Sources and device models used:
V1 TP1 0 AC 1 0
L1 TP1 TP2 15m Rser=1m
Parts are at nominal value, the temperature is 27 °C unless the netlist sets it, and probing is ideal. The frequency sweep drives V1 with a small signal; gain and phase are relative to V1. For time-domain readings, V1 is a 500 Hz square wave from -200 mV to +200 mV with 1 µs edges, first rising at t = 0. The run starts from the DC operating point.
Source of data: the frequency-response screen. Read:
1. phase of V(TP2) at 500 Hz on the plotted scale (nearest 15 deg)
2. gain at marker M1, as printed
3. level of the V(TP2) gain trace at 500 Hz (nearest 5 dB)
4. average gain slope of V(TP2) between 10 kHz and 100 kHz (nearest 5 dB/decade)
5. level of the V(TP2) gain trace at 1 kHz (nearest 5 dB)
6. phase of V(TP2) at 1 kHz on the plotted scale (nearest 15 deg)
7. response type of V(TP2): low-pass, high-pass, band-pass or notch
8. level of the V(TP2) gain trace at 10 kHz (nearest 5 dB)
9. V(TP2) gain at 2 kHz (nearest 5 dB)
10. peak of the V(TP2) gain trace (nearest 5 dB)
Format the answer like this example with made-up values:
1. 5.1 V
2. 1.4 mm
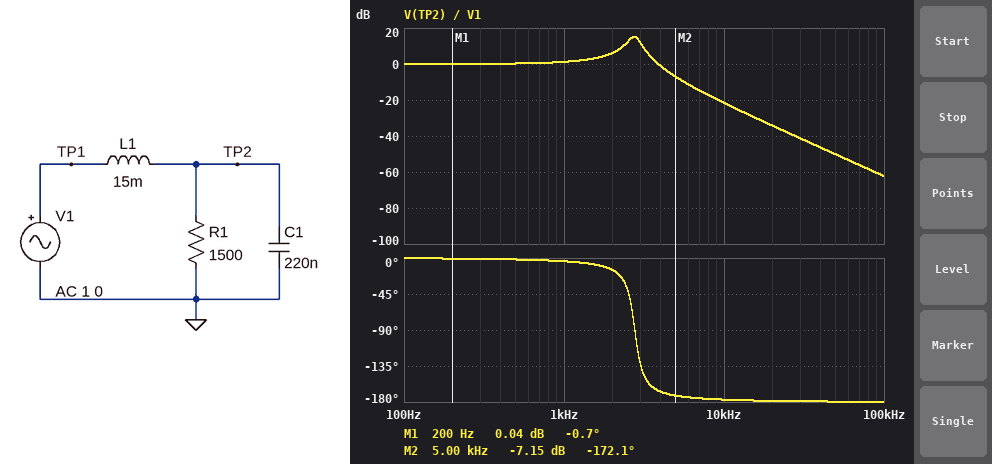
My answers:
1. 0 deg
2. 0.04 dB
3. 0 dB
4. -40 dB/decade
5. 0 dB
6. 0 deg
7. low-pass
8. -20 dB
9. 5 dB
10. 15 dB
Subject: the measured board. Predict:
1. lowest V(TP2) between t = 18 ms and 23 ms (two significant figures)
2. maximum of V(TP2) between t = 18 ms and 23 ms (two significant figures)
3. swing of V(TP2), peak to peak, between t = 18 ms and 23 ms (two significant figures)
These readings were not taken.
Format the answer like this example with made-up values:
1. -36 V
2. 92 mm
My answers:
1. -500 mV
2. 500 mV
3. 1.0 V
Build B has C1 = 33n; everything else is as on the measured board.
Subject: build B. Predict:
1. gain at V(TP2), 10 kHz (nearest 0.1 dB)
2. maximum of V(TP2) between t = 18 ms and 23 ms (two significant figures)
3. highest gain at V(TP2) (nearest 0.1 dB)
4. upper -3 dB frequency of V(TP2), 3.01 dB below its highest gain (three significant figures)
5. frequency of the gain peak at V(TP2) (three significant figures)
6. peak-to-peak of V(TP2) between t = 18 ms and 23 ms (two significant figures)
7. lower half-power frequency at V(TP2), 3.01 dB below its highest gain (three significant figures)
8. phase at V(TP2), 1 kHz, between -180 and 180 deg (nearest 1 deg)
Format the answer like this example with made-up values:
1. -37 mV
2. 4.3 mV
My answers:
1. -1.2 dB
2. 390 mV
3. 7.2 dB
4. 8.27 kHz
5. 6.78 kHz
6. 790 mV
7. 4.86 kHz
8. -4 deg
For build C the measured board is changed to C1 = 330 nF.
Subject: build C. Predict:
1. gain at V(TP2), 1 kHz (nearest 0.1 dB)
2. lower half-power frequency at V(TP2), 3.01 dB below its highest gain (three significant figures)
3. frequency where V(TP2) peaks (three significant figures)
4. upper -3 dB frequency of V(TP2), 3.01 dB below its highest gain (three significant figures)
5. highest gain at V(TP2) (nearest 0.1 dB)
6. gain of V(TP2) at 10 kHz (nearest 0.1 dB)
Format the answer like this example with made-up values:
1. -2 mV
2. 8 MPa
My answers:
1. 1.9 dB
2. 2.08 kHz
3. 2.25 kHz
4. 2.41 kHz
5. 17.0 dB
6. -25.4 dB
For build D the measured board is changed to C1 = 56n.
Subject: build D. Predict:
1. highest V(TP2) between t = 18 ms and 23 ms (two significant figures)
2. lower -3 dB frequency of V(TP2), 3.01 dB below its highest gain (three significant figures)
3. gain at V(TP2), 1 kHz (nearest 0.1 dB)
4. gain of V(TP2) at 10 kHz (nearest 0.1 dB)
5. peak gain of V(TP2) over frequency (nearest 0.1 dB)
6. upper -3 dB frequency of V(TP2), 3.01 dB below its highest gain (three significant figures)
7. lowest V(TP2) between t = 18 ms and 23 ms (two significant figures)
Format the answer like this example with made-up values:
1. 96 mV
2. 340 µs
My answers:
1. 430 mV
2. 4.26 kHz
3. 0.3 dB
4. -7.6 dB
5. 9.4 dB
6. 6.21 kHz
7. -430 mV
